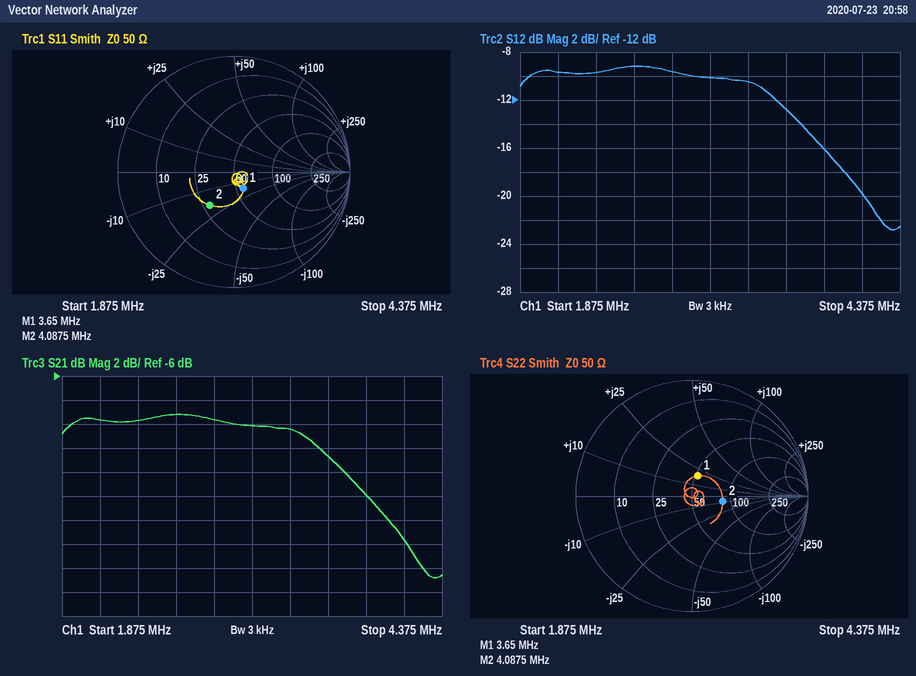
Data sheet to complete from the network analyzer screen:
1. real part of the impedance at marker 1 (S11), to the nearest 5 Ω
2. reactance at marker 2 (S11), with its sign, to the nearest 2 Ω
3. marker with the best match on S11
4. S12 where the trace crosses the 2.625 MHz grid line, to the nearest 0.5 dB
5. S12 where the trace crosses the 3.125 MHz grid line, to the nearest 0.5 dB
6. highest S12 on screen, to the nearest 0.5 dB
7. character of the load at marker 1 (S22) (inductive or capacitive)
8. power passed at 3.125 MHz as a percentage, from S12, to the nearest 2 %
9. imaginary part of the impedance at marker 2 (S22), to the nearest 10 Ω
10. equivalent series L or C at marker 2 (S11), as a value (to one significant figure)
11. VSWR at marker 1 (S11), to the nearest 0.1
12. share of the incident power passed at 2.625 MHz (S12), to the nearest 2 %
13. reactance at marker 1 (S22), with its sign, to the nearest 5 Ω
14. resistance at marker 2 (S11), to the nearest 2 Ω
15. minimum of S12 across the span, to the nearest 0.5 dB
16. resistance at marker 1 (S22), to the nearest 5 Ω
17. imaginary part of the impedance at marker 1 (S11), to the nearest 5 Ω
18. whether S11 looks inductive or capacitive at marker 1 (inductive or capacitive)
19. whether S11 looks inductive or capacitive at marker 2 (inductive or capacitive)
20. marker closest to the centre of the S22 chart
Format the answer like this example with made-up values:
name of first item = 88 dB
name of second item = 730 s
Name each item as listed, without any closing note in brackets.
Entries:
real part of the impedance at marker 1 (S11), to the nearest 5 Ω = 55 Ω
reactance at marker 2 (S11), with its sign, to the nearest 2 Ω = -18 Ω
marker with the best match on S11 = marker 1
S12 where the trace crosses the 2.625 MHz grid line, to the nearest 0.5 dB = -9.0 dB
S12 where the trace crosses the 3.125 MHz grid line, to the nearest 0.5 dB = -10.0 dB
highest S12 on screen, to the nearest 0.5 dB = -9.0 dB
character of the load at marker 1 (S22) = inductive
power passed at 3.125 MHz as a percentage, from S12, to the nearest 2 % = 10 %
imaginary part of the impedance at marker 2 (S22), to the nearest 10 Ω = -10 Ω
equivalent series L or C at marker 2 (S11), as a value = 2 nF
VSWR at marker 1 (S11), to the nearest 0.1 = 1.4
share of the incident power passed at 2.625 MHz (S12), to the nearest 2 % = 12 %
reactance at marker 1 (S22), with its sign, to the nearest 5 Ω = +20 Ω
resistance at marker 2 (S11), to the nearest 2 Ω = 28 Ω
minimum of S12 across the span, to the nearest 0.5 dB = -23.0 dB
resistance at marker 1 (S22), to the nearest 5 Ω = 50 Ω
imaginary part of the impedance at marker 1 (S11), to the nearest 5 Ω = -15 Ω
whether S11 looks inductive or capacitive at marker 1 = capacitive
whether S11 looks inductive or capacitive at marker 2 = capacitive
marker closest to the centre of the S22 chart = marker 1
